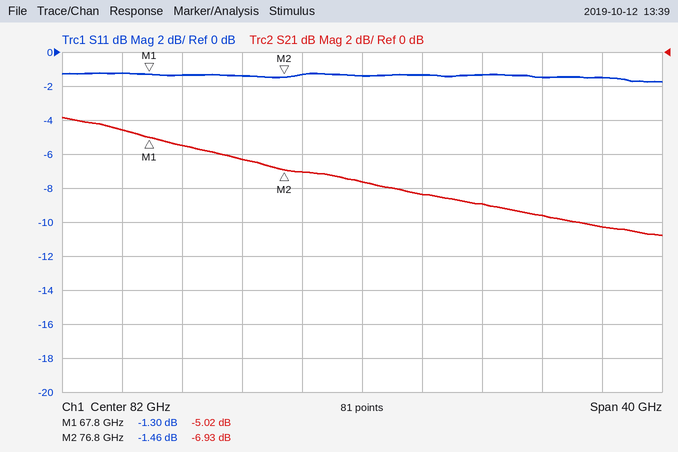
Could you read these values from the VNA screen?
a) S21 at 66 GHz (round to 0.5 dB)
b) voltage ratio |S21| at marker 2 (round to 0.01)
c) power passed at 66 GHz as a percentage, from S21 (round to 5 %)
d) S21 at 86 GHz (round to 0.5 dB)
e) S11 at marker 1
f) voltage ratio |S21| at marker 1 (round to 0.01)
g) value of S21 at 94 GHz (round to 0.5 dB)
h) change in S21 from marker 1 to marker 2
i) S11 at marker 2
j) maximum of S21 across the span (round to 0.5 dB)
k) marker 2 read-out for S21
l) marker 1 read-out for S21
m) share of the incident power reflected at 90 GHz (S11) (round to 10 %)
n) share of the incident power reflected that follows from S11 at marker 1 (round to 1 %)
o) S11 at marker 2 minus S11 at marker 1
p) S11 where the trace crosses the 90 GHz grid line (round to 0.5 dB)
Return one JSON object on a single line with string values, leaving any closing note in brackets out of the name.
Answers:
{"S21 at 66 GHz": "-4.5 dB", "voltage ratio |S21| at marker 2": "0.45", "power passed at 66 GHz as a percentage, from S21": "35 %", "S21 at 86 GHz": "-8.5 dB", "S11 at marker 1": "-1.30 dB", "voltage ratio |S21| at marker 1": "0.56", "value of S21 at 94 GHz": "-9.5 dB", "change in S21 from marker 1 to marker 2": "-1.91 dB", "S11 at marker 2": "-1.46 dB", "maximum of S21 across the span": "-4.0 dB", "marker 2 read-out for S21": "-6.93 dB", "marker 1 read-out for S21": "-5.02 dB", "share of the incident power reflected at 90 GHz (S11)": "70 %", "share of the incident power reflected that follows from S11 at marker 1": "74 %", "S11 at marker 2 minus S11 at marker 1": "-0.16 dB", "S11 where the trace crosses the 90 GHz grid line": "-1.5 dB"}
